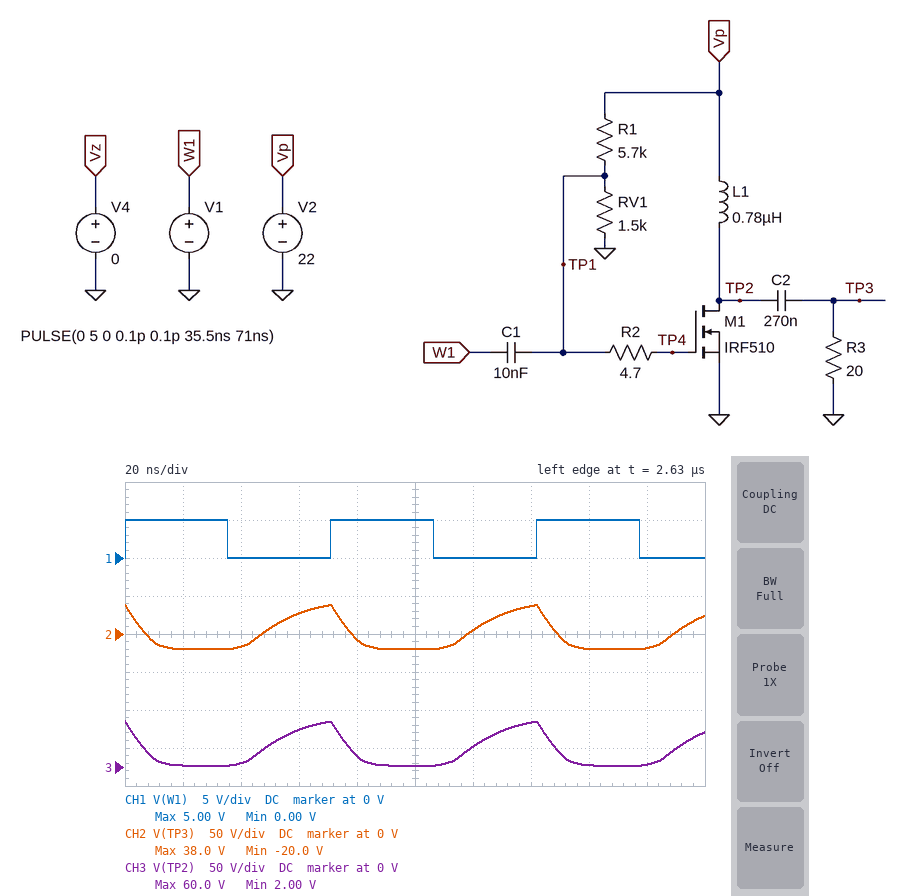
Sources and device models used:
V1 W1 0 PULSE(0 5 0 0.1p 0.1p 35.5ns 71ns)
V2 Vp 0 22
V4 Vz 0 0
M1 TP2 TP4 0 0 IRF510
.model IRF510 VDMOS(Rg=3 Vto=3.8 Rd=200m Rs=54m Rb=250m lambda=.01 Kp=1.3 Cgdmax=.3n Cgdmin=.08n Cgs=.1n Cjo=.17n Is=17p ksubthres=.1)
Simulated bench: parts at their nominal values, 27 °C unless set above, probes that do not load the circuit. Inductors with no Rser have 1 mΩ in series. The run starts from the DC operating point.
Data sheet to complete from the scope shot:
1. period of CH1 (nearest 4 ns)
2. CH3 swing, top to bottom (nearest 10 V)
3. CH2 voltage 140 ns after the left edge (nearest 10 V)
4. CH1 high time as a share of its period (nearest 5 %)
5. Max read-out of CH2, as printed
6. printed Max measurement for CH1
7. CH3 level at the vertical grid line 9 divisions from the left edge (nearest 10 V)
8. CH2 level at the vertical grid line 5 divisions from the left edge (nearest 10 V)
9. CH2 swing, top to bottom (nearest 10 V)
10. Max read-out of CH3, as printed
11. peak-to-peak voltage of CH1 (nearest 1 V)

72 ns
60 V
40 V
50 %
38.0 V
5.00 V
0 V
-20 V
60 V
60.0 V
5 V
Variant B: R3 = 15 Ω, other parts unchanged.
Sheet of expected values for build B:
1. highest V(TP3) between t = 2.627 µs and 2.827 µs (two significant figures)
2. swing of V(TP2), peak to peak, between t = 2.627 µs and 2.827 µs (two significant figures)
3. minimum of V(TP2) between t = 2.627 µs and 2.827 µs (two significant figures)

36 V
55 V
2.1 V
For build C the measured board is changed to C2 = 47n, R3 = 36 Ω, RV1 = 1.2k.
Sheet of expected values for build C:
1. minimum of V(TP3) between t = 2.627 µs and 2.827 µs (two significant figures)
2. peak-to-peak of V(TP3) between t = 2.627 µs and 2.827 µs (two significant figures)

-21 V
59 V
